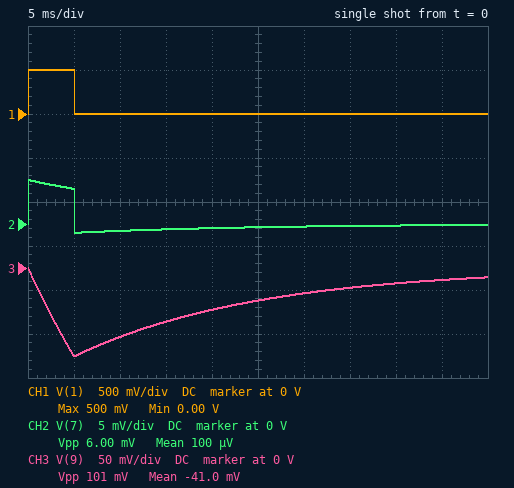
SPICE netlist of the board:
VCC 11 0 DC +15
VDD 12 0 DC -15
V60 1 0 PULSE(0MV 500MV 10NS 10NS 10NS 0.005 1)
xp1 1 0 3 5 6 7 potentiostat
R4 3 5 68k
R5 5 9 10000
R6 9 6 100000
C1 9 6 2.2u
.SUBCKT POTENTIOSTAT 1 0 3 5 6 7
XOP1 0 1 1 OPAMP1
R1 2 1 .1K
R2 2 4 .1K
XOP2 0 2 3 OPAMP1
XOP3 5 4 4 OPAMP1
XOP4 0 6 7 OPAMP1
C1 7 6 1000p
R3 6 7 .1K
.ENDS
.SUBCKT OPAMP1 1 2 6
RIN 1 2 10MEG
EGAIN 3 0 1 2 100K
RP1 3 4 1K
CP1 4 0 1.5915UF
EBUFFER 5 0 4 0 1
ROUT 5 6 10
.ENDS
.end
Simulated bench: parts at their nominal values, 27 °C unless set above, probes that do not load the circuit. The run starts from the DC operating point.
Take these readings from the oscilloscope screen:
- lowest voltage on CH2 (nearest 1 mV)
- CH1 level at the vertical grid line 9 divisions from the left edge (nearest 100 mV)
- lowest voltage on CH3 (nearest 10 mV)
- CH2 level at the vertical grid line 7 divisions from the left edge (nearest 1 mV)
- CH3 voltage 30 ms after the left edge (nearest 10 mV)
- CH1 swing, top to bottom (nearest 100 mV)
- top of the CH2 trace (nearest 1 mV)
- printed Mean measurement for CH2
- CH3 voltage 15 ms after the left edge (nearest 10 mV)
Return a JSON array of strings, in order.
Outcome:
["-1 mV", "0 V", "-100 mV", "0 V", "-30 mV", "500 mV", "5 mV", "100 µV", "-60 mV"]
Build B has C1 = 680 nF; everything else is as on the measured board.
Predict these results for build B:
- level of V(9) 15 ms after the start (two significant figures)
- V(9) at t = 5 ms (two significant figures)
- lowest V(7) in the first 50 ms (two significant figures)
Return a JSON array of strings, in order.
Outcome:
["-50 mV", "-250 mV", "-2.5 mV"]
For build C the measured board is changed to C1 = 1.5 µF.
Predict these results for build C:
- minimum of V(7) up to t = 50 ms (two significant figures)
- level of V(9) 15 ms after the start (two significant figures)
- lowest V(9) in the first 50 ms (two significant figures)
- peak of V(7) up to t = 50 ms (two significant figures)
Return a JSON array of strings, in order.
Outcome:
["-1.4 mV", "-67 mV", "-140 mV", "5.0 mV"]
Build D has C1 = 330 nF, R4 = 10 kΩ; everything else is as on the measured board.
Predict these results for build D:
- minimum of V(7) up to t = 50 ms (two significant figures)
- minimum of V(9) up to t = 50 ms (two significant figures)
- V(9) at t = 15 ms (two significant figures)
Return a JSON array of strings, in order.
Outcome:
["-3.7 mV", "-370 mV", "-13 mV"]
